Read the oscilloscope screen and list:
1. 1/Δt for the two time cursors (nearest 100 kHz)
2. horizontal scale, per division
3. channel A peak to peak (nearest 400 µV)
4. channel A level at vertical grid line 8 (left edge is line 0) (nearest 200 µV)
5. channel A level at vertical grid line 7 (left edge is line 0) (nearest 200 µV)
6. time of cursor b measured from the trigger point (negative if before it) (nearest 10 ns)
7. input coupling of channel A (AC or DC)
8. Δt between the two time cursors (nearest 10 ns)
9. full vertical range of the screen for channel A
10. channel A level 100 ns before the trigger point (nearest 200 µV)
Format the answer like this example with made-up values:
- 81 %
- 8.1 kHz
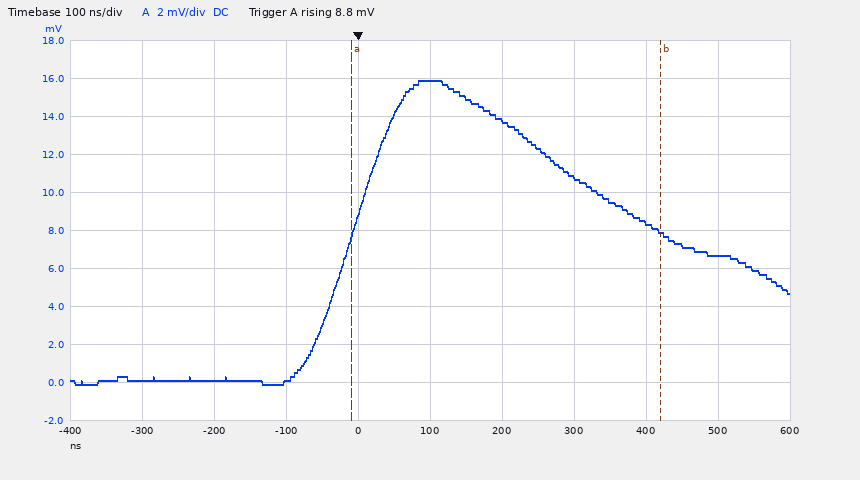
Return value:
- 2.3 MHz
- 100 ns
- 16.0 mV
- 8.4 mV
- 10.8 mV
- +420 ns
- DC
- 430 ns
- 20 mV
- 0.0 mV
